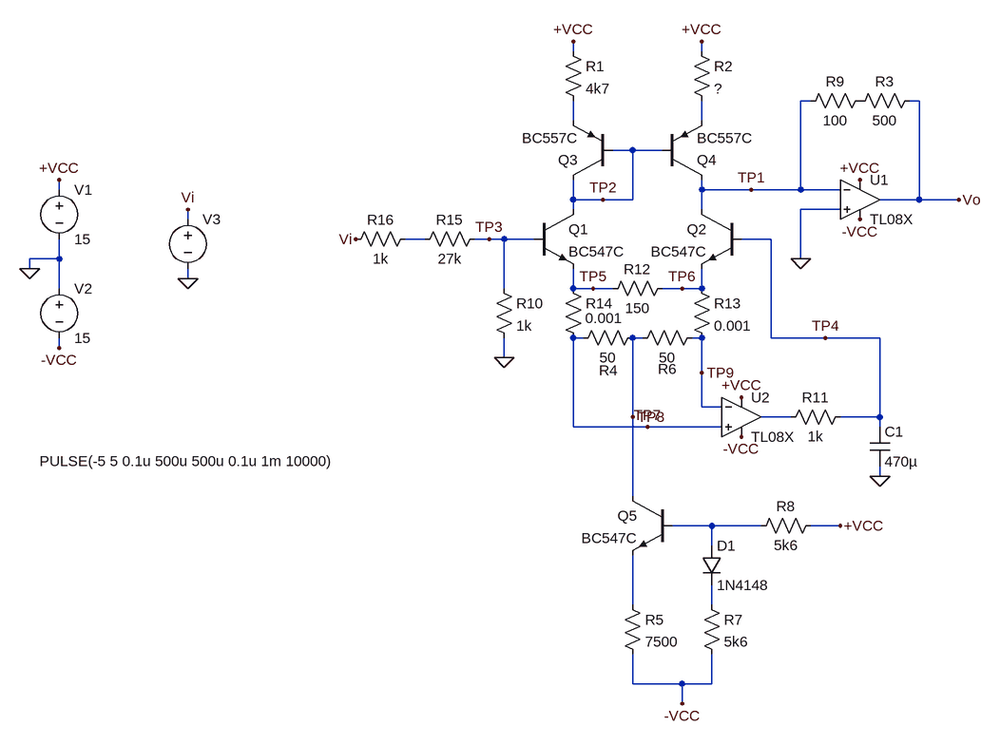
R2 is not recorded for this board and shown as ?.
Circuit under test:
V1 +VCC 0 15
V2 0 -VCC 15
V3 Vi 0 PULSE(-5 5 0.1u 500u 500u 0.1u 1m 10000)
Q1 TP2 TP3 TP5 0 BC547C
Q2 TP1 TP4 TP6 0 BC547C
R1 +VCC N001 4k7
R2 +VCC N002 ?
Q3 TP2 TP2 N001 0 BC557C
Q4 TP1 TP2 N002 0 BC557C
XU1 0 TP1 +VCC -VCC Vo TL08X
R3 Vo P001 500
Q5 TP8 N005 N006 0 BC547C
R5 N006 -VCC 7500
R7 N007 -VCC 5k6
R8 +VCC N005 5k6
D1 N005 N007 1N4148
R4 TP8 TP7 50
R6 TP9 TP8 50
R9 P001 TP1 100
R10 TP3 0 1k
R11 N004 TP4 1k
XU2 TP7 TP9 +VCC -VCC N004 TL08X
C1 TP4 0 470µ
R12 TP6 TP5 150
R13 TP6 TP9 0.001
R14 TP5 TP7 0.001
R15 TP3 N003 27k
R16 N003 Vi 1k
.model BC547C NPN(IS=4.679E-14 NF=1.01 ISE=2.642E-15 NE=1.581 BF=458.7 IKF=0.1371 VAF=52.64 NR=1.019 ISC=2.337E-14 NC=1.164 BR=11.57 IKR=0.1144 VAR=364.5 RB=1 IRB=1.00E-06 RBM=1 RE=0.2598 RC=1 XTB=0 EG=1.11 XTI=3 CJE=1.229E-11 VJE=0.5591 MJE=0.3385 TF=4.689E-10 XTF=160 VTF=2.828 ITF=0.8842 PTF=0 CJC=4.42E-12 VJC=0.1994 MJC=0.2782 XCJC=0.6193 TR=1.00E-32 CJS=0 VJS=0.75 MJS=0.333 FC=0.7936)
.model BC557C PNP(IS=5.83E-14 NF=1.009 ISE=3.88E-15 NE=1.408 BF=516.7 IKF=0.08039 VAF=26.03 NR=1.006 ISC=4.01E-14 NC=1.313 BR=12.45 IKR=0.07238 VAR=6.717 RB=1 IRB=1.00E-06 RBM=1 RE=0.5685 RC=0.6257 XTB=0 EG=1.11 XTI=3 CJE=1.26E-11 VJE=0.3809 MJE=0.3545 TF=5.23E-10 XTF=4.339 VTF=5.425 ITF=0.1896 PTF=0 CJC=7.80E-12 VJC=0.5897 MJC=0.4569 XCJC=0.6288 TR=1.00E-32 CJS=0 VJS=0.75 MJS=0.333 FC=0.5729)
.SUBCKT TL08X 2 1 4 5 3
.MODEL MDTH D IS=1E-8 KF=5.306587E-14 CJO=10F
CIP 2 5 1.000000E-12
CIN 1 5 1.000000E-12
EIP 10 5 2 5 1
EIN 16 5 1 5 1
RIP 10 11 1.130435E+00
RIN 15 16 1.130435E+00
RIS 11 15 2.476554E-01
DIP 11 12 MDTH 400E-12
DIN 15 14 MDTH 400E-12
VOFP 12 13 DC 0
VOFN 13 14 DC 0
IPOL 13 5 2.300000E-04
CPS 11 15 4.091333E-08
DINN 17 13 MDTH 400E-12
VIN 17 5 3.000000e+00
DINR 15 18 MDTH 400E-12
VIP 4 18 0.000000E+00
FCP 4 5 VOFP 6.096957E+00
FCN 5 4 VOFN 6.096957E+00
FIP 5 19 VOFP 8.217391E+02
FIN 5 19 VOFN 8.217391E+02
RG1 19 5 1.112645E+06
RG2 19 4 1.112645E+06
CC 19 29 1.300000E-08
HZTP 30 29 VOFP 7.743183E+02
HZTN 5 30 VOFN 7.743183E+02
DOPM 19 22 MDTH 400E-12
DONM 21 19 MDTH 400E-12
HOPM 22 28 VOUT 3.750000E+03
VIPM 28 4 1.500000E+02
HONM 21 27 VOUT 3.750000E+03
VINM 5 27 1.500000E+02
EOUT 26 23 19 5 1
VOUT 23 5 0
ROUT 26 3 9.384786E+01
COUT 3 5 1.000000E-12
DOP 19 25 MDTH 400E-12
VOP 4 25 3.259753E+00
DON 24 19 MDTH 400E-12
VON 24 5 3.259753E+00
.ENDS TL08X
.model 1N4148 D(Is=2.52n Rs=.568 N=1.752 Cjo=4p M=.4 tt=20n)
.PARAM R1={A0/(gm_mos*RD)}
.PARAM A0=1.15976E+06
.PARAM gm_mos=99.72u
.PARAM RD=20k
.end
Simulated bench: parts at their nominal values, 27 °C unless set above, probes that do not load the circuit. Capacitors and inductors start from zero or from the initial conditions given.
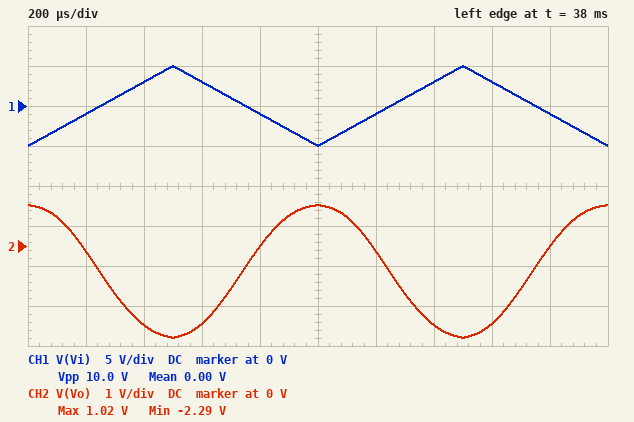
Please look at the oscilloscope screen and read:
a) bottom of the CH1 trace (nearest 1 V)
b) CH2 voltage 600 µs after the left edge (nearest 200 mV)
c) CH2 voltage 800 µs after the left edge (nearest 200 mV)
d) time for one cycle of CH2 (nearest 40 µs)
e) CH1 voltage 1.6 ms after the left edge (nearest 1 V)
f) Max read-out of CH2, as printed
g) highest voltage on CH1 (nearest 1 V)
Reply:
-5 V
-2.0 V
0 V
1.00 ms
3 V
1.02 V
5 V
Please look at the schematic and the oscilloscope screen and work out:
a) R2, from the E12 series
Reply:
2.2 kΩ
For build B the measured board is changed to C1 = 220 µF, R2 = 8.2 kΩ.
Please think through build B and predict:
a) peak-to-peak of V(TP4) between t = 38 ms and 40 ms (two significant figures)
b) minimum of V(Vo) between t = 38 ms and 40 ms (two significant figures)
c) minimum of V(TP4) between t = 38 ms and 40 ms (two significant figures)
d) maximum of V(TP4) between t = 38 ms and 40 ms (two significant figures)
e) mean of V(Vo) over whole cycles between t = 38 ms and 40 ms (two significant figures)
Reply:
25 mV
-610 mV
-9.4 mV
15 mV
220 mV
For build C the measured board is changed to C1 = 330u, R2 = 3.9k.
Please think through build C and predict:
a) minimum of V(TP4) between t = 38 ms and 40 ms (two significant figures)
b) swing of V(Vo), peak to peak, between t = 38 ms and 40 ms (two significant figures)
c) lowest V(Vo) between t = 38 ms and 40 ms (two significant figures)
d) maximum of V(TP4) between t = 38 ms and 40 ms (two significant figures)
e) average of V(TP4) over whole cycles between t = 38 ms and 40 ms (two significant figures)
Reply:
-5.2 mV
2.3 V
-1.3 V
11 mV
3.0 mV
